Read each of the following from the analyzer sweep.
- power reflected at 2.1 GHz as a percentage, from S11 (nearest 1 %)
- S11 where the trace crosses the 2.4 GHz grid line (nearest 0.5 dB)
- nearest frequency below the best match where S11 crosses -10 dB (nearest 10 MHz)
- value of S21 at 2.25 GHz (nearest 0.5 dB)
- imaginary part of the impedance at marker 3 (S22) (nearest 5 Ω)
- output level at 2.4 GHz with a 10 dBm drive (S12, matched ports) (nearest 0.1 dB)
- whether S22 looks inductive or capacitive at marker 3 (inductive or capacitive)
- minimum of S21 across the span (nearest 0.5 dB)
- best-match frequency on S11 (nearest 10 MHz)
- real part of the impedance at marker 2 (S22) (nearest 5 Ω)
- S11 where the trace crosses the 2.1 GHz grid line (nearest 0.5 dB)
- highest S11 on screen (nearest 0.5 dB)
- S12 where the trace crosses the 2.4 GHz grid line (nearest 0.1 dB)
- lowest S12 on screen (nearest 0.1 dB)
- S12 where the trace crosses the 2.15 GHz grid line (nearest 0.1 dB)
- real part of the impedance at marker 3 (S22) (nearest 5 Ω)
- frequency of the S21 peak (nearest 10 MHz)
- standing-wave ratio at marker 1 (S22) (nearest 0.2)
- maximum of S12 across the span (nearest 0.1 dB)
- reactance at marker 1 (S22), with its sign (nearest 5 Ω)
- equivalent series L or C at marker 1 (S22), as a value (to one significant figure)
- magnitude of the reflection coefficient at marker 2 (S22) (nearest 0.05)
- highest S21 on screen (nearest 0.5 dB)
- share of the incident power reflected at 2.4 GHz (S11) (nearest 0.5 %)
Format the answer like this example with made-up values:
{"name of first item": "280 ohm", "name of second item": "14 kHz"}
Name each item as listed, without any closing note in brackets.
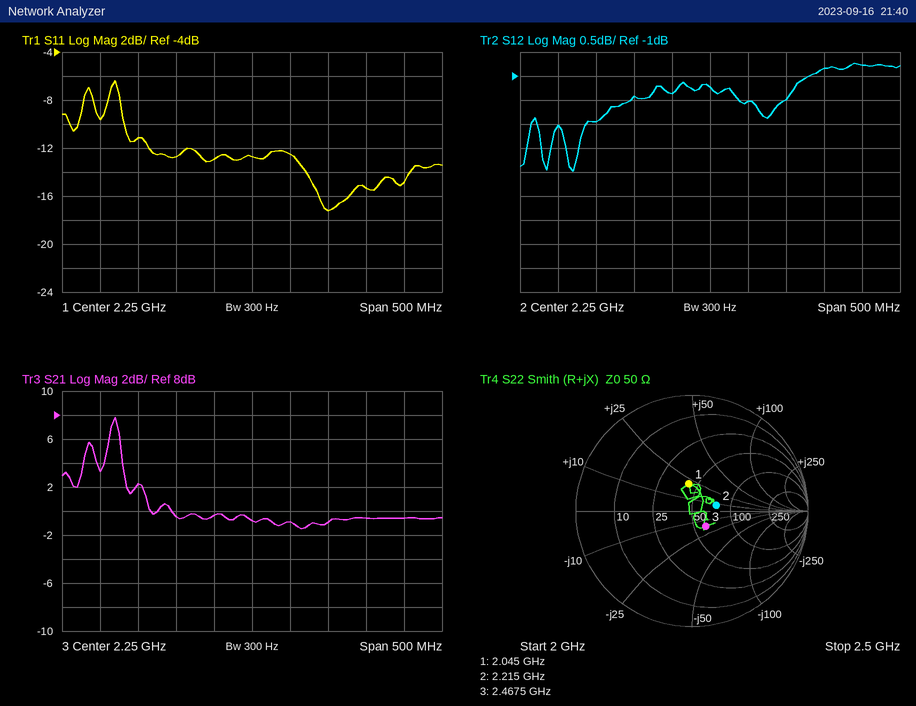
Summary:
{"power reflected at 2.1 GHz as a percentage, from S11": "8 %", "S11 where the trace crosses the 2.4 GHz grid line": "-15.5 dB", "nearest frequency below the best match where S11 crosses -10 dB": "2.08 GHz", "value of S21 at 2.25 GHz": "-1.0 dB", "imaginary part of the impedance at marker 3 (S22)": "-15 Ω", "output level at 2.4 GHz with a 10 dBm drive (S12, matched ports)": "9.2 dBm", "whether S22 looks inductive or capacitive at marker 3": "capacitive", "minimum of S21 across the span": "-1.5 dB", "best-match frequency on S11": "2.35 GHz", "real part of the impedance at marker 2 (S22)": "75 Ω", "S11 where the trace crosses the 2.1 GHz grid line": "-11.0 dB", "highest S11 on screen": "-6.5 dB", "S12 where the trace crosses the 2.4 GHz grid line": "-0.8 dB", "lowest S12 on screen": "-3.0 dB", "S12 where the trace crosses the 2.15 GHz grid line": "-1.4 dB", "real part of the impedance at marker 3 (S22)": "60 Ω", "frequency of the S21 peak": "2.07 GHz", "standing-wave ratio at marker 1 (S22)": "1.6", "maximum of S12 across the span": "-0.7 dB", "reactance at marker 1 (S22), with its sign": "+20 Ω", "equivalent series L or C at marker 1 (S22), as a value": "2 nH", "magnitude of the reflection coefficient at marker 2 (S22)": "0.20", "highest S21 on screen": "8.0 dB", "share of the incident power reflected at 2.4 GHz (S11)": "3.0 %"}
